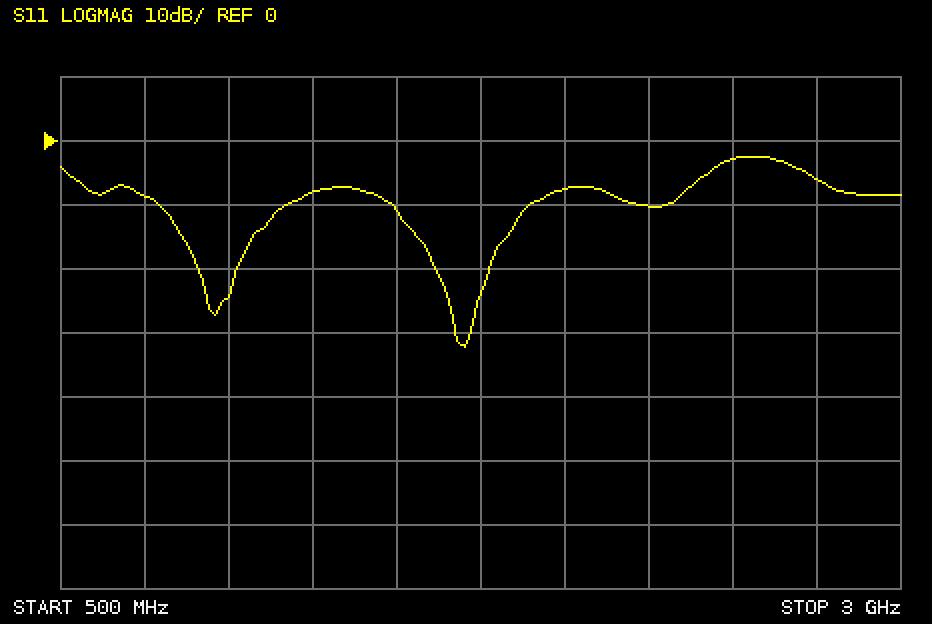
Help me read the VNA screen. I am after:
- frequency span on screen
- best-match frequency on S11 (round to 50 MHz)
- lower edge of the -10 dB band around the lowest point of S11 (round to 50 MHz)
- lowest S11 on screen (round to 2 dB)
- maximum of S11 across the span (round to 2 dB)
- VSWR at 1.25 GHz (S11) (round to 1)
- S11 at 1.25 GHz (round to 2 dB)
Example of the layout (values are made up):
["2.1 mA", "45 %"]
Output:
["2.5 GHz", "1.70 GHz", "1.50 GHz", "-32 dB", "-2 dB", "2", "-8 dB"]
